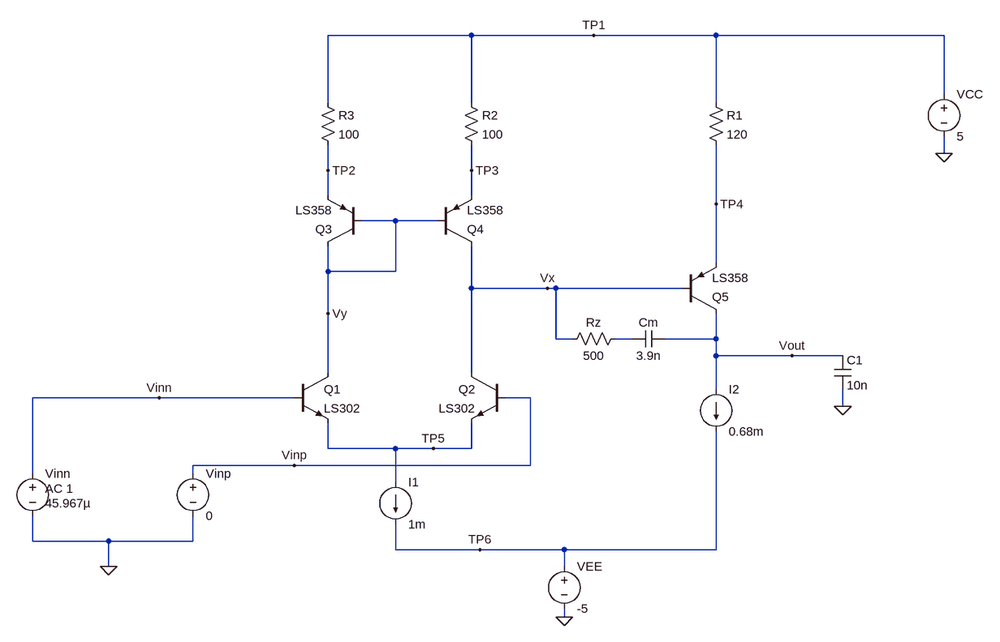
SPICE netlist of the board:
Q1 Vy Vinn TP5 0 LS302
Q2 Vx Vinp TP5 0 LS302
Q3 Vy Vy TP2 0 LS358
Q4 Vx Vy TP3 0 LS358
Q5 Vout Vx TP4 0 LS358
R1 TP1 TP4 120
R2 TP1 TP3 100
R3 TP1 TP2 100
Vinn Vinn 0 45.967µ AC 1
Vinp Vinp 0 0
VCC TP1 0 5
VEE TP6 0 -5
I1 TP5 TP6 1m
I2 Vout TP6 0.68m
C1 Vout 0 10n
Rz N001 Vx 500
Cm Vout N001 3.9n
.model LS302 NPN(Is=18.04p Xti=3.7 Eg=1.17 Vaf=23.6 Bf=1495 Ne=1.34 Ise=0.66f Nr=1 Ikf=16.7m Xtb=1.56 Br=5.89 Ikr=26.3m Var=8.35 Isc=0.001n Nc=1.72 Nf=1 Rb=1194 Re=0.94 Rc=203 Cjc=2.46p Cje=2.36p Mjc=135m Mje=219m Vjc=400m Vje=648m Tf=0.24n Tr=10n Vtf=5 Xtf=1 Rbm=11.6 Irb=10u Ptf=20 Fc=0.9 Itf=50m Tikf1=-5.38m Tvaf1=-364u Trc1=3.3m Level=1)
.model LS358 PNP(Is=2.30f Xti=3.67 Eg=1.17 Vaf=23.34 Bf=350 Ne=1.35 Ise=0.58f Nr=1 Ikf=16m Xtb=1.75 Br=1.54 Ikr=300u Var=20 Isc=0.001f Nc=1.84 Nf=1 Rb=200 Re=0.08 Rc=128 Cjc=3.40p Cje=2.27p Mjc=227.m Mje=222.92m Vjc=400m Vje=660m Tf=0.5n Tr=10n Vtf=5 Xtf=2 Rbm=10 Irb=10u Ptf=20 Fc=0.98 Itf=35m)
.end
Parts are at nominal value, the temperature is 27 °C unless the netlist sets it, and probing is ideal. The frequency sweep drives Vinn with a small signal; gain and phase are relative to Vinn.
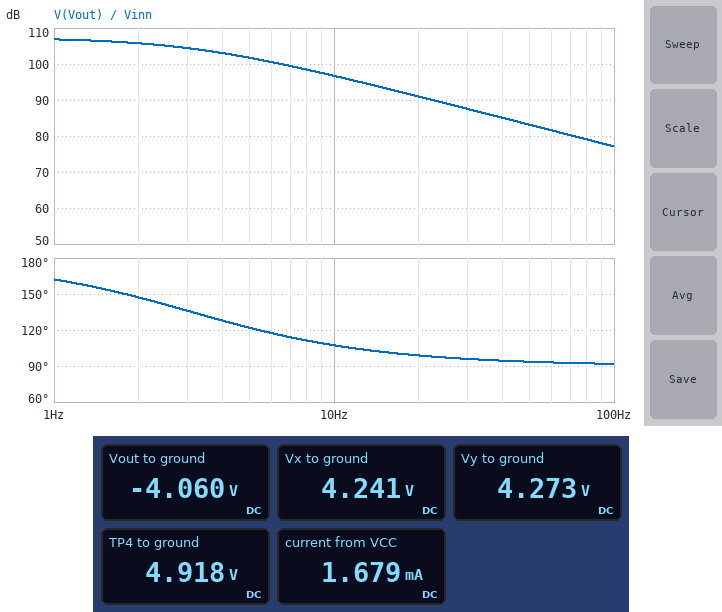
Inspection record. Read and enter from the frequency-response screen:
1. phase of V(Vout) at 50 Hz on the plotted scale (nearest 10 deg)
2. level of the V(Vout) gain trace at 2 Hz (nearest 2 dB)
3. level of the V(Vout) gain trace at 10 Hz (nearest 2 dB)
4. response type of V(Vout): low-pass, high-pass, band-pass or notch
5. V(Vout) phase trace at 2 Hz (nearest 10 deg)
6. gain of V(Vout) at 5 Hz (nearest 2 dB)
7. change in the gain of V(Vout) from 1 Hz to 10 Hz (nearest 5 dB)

90 deg
106 dB
96 dB
low-pass
150 deg
102 dB
-10 dB
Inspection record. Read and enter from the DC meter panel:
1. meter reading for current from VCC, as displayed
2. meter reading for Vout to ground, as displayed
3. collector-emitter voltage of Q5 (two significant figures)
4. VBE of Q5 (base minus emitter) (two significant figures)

1.679 mA
-4.060 V
-9.0 V
-680 mV
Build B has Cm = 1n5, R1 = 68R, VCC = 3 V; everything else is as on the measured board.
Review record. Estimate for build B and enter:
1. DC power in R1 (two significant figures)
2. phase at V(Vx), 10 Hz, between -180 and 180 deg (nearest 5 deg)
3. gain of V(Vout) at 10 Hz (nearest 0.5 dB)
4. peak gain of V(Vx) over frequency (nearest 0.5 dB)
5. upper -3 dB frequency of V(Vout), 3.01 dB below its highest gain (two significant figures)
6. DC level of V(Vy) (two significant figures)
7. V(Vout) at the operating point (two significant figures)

32 µW
-5 deg
85.0 dB
29.0 dB
100 Hz
2.3 V
2.6 V
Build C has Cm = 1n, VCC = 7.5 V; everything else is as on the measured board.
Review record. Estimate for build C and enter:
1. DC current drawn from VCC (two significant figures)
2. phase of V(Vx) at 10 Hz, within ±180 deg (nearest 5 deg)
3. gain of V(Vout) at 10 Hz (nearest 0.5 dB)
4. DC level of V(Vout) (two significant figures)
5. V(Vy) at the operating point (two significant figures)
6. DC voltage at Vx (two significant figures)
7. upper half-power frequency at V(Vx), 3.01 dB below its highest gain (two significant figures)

1.7 mA
-35 deg
105.0 dB
-950 mV
6.8 V
6.7 V
12 Hz
